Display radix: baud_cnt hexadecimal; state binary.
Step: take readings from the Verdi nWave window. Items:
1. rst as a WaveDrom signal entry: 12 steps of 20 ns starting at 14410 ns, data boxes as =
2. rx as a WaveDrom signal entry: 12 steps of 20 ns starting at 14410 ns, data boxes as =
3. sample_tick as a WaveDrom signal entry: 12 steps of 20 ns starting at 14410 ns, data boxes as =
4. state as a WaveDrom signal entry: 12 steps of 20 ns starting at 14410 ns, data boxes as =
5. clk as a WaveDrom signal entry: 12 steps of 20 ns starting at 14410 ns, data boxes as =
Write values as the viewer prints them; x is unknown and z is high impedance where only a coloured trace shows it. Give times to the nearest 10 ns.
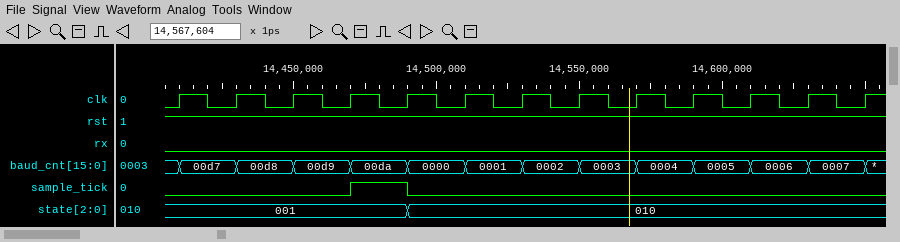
{name: 'rst', wave: '1...........'}
{name: 'rx', wave: '0...........'}
{name: 'sample_tick', wave: '0..10.......'}
{name: 'state', wave: '=...=.......', data: '001 010'}
{name: 'clk', wave: 'p...........'}
